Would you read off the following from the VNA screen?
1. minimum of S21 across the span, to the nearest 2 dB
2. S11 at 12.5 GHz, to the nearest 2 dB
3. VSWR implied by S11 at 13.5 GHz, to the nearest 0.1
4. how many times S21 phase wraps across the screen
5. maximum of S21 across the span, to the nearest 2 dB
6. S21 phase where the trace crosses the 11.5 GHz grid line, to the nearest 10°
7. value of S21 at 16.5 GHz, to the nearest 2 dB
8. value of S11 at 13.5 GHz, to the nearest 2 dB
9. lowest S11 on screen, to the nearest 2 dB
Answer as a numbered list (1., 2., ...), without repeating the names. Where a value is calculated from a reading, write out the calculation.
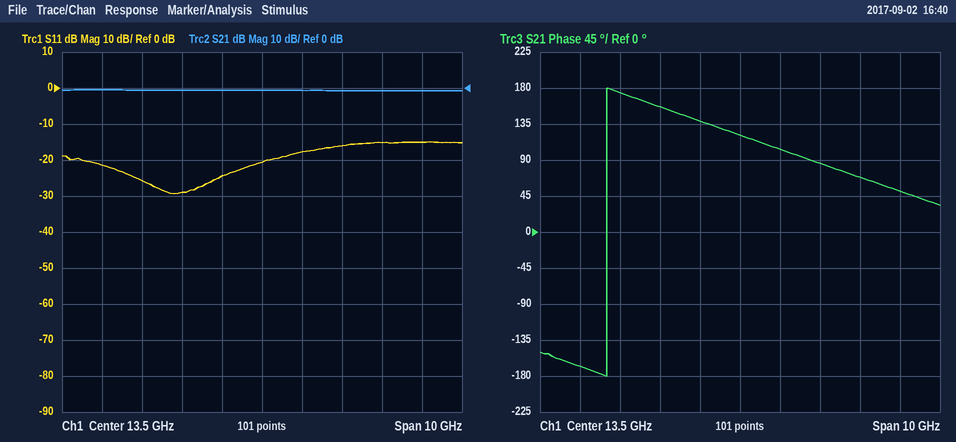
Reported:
1. 0 dB
2. -24 dB
3. |Γ| = 10^(-20/20) = 0.1000; VSWR = (1 + 0.1000)/(1 − 0.1000) ≈ 1.2
4. 1
5. 0 dB
6. 160°
7. 0 dB
8. -20 dB
9. -30 dB
